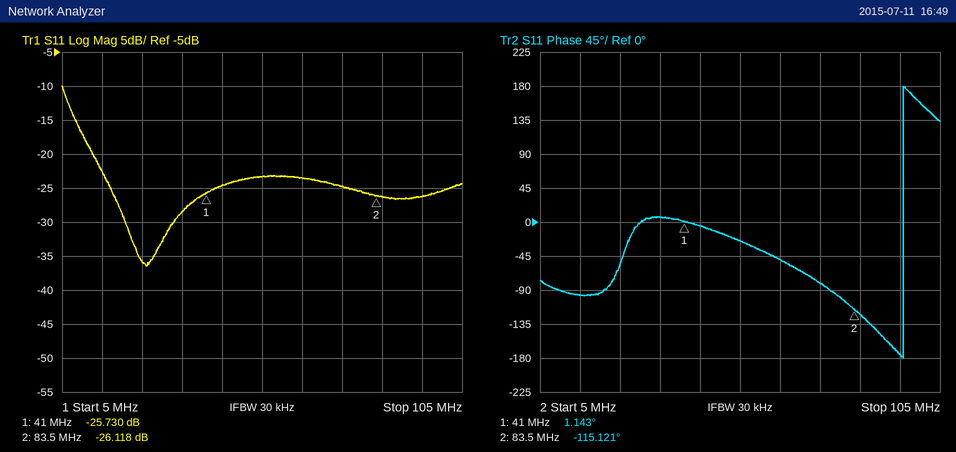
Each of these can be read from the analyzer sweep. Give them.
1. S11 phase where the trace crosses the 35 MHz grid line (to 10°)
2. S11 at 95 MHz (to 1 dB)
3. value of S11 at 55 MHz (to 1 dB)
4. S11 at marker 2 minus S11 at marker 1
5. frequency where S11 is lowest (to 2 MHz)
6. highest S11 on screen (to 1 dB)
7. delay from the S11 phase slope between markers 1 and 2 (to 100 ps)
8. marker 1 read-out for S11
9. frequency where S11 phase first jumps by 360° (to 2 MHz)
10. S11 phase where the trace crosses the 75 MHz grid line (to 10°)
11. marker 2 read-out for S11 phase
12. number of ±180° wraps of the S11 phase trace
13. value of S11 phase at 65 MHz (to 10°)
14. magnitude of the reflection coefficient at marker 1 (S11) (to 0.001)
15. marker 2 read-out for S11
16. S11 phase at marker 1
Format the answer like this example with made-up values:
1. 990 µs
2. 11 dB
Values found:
1. 10°
2. -26 dB
3. -23 dB
4. -0.388 dB
5. 26 MHz
6. -10 dB
7. 7.6 ns
8. -25.730 dB
9. 96 MHz
10. -80°
11. -115.121°
12. 1
13. -50°
14. 0.052
15. -26.118 dB
16. 1.143°
